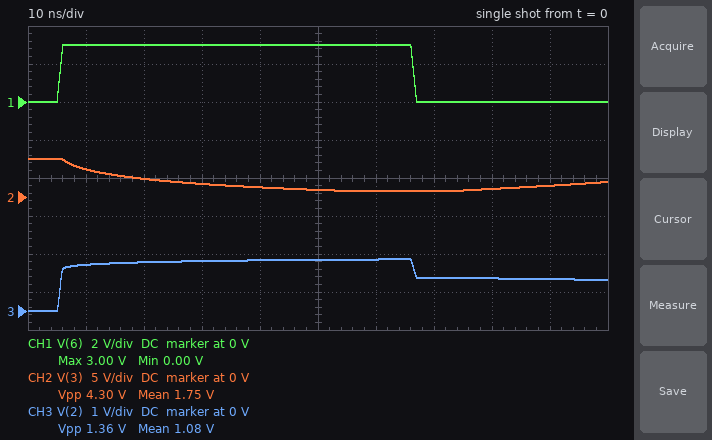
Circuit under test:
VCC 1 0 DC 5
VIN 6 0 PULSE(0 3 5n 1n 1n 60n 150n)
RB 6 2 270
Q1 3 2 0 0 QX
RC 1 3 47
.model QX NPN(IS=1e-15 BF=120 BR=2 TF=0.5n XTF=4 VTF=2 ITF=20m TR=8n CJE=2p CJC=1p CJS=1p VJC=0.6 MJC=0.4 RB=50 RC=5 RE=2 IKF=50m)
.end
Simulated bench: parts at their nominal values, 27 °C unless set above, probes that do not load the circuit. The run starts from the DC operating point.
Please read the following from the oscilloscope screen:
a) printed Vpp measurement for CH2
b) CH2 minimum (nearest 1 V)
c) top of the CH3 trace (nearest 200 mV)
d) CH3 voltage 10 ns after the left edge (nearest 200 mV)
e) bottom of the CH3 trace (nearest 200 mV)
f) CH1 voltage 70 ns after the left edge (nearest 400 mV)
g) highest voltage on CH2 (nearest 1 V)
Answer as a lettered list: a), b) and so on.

a) 4.30 V
b) 1 V
c) 1.4 V
d) 1.2 V
e) 0 V
f) 0 V
g) 5 V
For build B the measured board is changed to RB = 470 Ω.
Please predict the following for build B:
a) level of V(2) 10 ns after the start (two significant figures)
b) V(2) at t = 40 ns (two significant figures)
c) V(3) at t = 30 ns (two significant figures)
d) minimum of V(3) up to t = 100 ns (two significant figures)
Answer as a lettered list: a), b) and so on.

a) 1.1 V
b) 1.2 V
c) 2.4 V
d) 1.3 V
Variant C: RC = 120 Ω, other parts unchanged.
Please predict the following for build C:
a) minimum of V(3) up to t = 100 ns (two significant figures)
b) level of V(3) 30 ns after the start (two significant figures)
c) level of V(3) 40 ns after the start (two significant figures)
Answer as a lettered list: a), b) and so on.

a) 320 mV
b) 360 mV
c) 350 mV
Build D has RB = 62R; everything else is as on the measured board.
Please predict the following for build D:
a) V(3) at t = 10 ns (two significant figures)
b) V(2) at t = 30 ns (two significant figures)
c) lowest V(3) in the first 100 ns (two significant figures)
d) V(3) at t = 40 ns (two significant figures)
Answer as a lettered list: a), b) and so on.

a) 2.5 V
b) 1.9 V
c) 690 mV
d) 750 mV
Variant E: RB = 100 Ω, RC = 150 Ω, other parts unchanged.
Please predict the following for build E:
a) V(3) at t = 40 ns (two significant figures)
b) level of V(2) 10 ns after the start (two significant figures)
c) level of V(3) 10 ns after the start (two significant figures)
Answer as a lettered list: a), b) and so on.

a) 290 mV
b) 1.6 V
c) 460 mV
